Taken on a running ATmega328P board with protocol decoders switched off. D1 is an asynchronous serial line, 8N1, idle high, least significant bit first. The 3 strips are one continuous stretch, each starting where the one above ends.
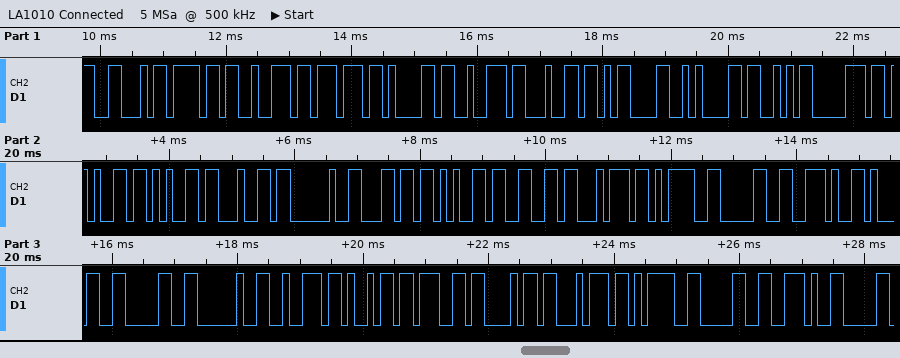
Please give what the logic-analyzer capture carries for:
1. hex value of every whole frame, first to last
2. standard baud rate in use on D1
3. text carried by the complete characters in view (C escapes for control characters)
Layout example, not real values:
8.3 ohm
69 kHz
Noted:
0x46 0x6F 0x72 0x77 0x61 0x72 0x64 0x0D 0x0A 0x53 0x70 0x65 0x65 0x64 0x20 0x6C 0x65 0x66 0x74 0x3D 0x30 0x2E 0x31 0x30 0x20 0x72 0x69 0x67 0x68 0x74 0x3D 0x30 0x2E
9600 baud
"Forward\r\nSpeed left=0.10 right=0."
